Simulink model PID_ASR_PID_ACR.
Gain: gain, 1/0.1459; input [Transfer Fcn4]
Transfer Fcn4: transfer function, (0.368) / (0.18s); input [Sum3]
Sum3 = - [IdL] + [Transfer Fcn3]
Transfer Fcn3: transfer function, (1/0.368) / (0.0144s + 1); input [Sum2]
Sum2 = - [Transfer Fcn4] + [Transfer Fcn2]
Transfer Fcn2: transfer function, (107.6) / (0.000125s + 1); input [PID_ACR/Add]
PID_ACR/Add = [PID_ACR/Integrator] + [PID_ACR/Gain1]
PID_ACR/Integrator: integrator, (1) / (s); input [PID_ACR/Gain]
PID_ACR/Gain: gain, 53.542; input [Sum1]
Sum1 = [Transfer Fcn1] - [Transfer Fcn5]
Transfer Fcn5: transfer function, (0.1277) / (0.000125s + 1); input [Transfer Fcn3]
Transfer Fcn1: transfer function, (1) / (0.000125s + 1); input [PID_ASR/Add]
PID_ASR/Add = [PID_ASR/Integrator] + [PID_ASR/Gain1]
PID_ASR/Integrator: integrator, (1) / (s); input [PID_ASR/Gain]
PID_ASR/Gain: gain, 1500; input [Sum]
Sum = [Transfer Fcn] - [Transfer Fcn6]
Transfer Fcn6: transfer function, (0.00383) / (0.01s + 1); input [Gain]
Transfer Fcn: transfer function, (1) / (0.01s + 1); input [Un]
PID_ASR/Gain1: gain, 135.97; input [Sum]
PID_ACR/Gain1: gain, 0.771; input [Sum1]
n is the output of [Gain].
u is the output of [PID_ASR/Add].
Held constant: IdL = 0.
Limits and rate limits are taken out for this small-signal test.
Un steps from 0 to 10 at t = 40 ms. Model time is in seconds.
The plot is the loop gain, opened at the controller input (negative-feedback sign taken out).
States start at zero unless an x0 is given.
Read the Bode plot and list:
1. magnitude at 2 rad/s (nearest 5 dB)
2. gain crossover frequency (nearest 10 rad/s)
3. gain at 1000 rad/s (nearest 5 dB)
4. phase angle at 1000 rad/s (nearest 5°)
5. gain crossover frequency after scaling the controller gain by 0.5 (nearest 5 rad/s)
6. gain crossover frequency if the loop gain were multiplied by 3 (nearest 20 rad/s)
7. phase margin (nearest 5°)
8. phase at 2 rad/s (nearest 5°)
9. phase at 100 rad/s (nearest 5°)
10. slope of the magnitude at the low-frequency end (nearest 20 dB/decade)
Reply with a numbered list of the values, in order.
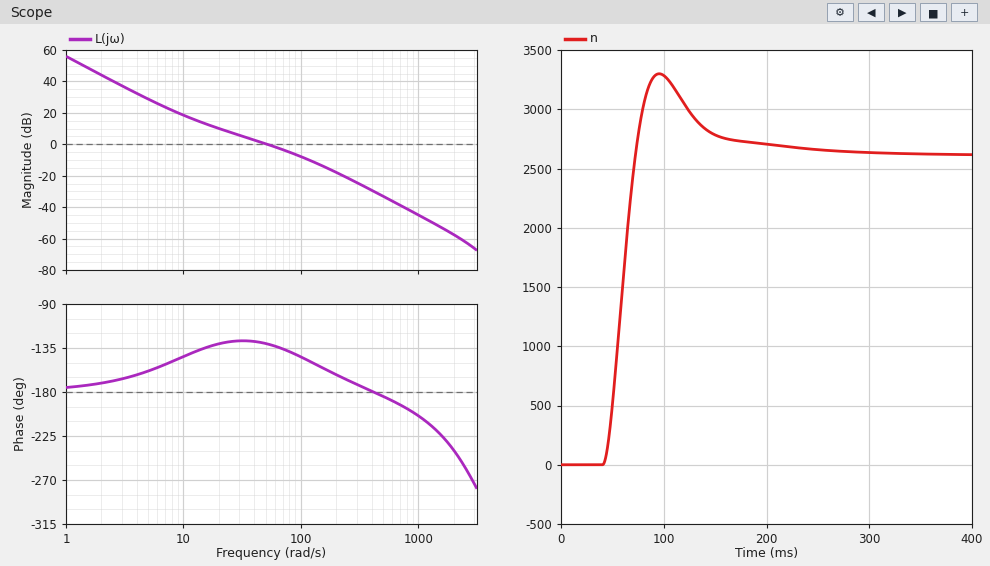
1. 45 dB
2. 50 rad/s
3. -45 dB
4. -205°
5. 30 rad/s
6. 120 rad/s
7. 50°
8. -170°
9. -145°
10. -40 dB/decade
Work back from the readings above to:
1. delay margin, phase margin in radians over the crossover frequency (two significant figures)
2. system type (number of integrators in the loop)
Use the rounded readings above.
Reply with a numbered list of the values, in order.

1. 0.017 s
2. 2
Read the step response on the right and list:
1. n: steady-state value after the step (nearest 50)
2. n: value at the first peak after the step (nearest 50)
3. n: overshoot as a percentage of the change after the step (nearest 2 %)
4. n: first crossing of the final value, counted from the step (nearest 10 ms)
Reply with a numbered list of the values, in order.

1. 2600
2. 3300
3. 26 %
4. 30 ms
